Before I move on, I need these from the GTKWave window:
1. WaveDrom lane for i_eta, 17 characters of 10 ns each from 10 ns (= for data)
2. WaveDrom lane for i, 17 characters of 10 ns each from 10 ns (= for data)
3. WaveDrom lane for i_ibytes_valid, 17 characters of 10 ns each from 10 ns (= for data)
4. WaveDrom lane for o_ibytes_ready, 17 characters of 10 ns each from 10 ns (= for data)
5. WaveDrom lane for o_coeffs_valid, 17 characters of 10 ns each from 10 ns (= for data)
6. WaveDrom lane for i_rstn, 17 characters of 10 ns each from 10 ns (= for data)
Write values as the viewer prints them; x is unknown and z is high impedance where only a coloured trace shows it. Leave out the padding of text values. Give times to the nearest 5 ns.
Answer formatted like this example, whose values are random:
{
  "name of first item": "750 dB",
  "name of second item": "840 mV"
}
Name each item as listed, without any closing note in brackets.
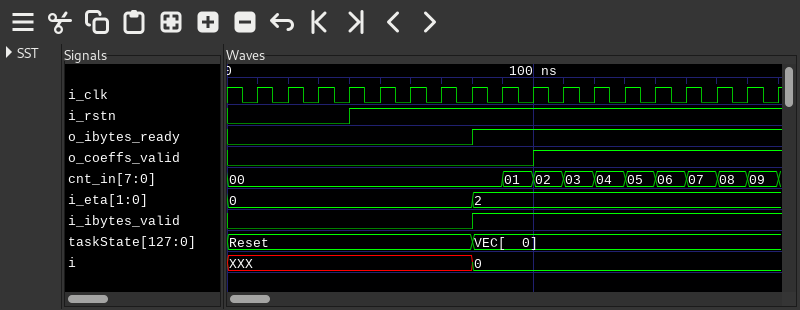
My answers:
{
  "WaveDrom lane for i_eta, 17 characters of 10 ns each from 10 ns": "{name: 'i_eta', wave: '=......=.........', data: '0 2'}",
  "WaveDrom lane for i, 17 characters of 10 ns each from 10 ns": "{name: 'i', wave: 'x......=.........', data: '0'}",
  "WaveDrom lane for i_ibytes_valid, 17 characters of 10 ns each from 10 ns": "{name: 'i_ibytes_valid', wave: '0......1.........'}",
  "WaveDrom lane for o_ibytes_ready, 17 characters of 10 ns each from 10 ns": "{name: 'o_ibytes_ready', wave: '0......1.........'}",
  "WaveDrom lane for o_coeffs_valid, 17 characters of 10 ns each from 10 ns": "{name: 'o_coeffs_valid', wave: '0........1.......'}",
  "WaveDrom lane for i_rstn, 17 characters of 10 ns each from 10 ns": "{name: 'i_rstn', wave: '0..1.............'}"
}
